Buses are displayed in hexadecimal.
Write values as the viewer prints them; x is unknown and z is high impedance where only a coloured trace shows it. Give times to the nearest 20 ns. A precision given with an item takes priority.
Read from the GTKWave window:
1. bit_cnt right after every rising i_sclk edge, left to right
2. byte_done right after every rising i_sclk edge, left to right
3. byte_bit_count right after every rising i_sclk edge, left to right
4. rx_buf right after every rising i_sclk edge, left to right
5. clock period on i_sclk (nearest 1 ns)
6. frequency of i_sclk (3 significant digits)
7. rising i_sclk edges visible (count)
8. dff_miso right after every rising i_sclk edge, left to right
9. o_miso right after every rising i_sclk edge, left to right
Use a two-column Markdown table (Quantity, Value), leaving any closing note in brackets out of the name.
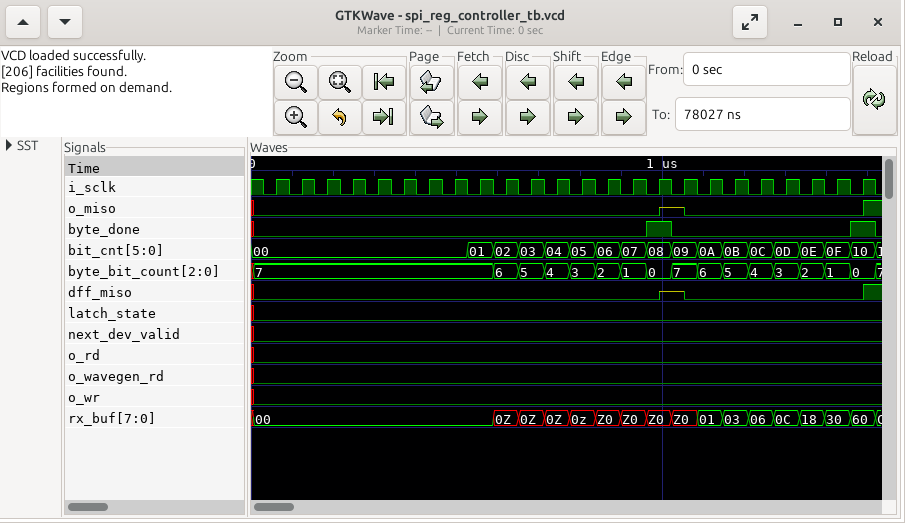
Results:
| Quantity | Value |
|---|---|
| bit_cnt right after every rising i_sclk edge, left to right | 00, 00, 00, 00, 00, 00, 00, 00, 01, 02, 03, 04, 05, 06, 07, 08, 09, 0A, 0B, 0C, 0D, 0E, 0F, 10 |
| byte_done right after every rising i_sclk edge, left to right | 0 0 0 0 0 0 0 0 0 0 0 0 0 0 0 1 0 0 0 0 0 0 0 1 |
| byte_bit_count right after every rising i_sclk edge, left to right | 7, 7, 7, 7, 7, 7, 7, 7, 7, 6, 5, 4, 3, 2, 1, 0, 7, 6, 5, 4, 3, 2, 1, 0 |
| rx_buf right after every rising i_sclk edge, left to right | 00, 00, 00, 00, 00, 00, 00, 00, 00, 0Z, 0Z, 0Z, 0z, Z0, Z0, Z0, Z0, 01, 03, 06, 0C, 18, 30, 60 |
| clock period on i_sclk | 62 ns |
| frequency of i_sclk | 16.1 MHz |
| rising i_sclk edges visible | 24 |
| dff_miso right after every rising i_sclk edge, left to right | 0 0 0 0 0 0 0 0 0 0 0 0 0 0 0 z 0 0 0 0 0 0 0 1 |
| o_miso right after every rising i_sclk edge, left to right | 0 0 0 0 0 0 0 0 0 0 0 0 0 0 0 z 0 0 0 0 0 0 0 1 |
